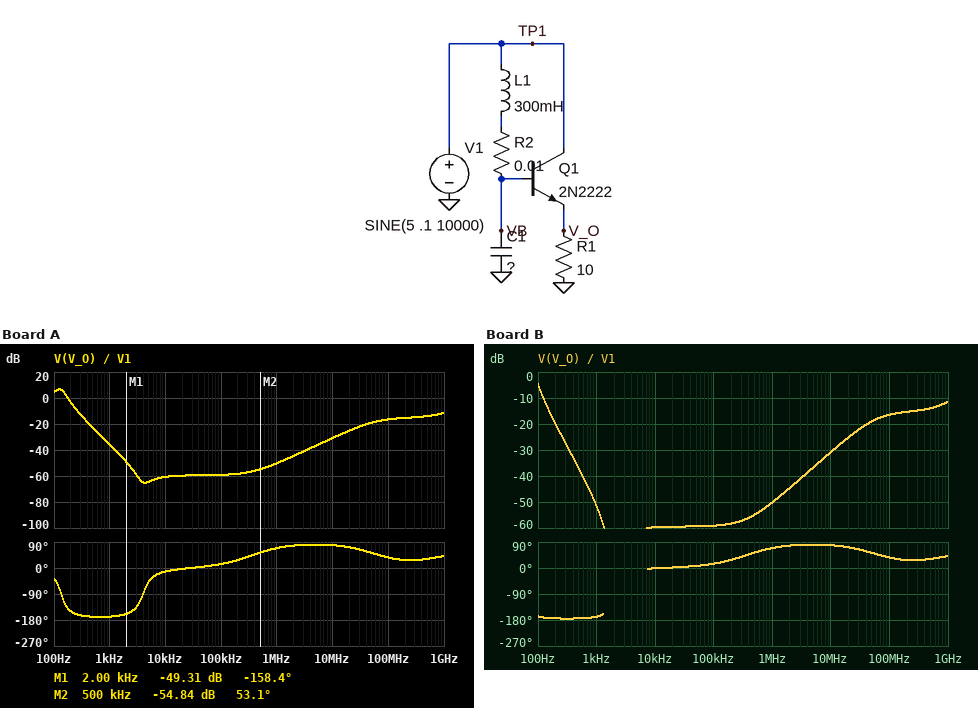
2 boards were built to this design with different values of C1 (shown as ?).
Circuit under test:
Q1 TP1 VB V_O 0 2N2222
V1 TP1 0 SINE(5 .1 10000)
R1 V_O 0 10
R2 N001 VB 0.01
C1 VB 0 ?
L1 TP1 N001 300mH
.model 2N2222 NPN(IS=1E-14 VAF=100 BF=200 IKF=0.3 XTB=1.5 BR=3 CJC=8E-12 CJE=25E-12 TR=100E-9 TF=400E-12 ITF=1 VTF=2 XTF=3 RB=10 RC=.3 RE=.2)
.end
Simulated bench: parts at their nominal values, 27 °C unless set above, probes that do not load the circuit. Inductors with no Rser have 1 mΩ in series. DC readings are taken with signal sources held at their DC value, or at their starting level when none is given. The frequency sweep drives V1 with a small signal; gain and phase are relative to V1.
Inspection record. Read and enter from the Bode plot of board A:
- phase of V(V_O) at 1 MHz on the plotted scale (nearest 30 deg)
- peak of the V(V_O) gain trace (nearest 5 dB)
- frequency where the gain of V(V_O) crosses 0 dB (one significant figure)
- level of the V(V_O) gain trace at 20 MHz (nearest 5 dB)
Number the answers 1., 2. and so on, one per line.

1. 60 deg
2. 5 dB
3. 200 Hz
4. -25 dB
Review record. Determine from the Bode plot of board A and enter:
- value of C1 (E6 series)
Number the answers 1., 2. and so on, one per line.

1. 4.7 µF
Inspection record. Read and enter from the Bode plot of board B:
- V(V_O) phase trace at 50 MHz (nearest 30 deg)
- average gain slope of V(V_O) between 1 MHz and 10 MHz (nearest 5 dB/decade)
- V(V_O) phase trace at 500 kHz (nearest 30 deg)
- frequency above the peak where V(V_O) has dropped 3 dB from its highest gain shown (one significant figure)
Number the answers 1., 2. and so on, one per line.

1. 60 deg
2. 20 dB/decade
3. 60 deg
4. 100 Hz
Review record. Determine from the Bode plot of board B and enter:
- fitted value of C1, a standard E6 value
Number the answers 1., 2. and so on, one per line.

1. 22 µF
